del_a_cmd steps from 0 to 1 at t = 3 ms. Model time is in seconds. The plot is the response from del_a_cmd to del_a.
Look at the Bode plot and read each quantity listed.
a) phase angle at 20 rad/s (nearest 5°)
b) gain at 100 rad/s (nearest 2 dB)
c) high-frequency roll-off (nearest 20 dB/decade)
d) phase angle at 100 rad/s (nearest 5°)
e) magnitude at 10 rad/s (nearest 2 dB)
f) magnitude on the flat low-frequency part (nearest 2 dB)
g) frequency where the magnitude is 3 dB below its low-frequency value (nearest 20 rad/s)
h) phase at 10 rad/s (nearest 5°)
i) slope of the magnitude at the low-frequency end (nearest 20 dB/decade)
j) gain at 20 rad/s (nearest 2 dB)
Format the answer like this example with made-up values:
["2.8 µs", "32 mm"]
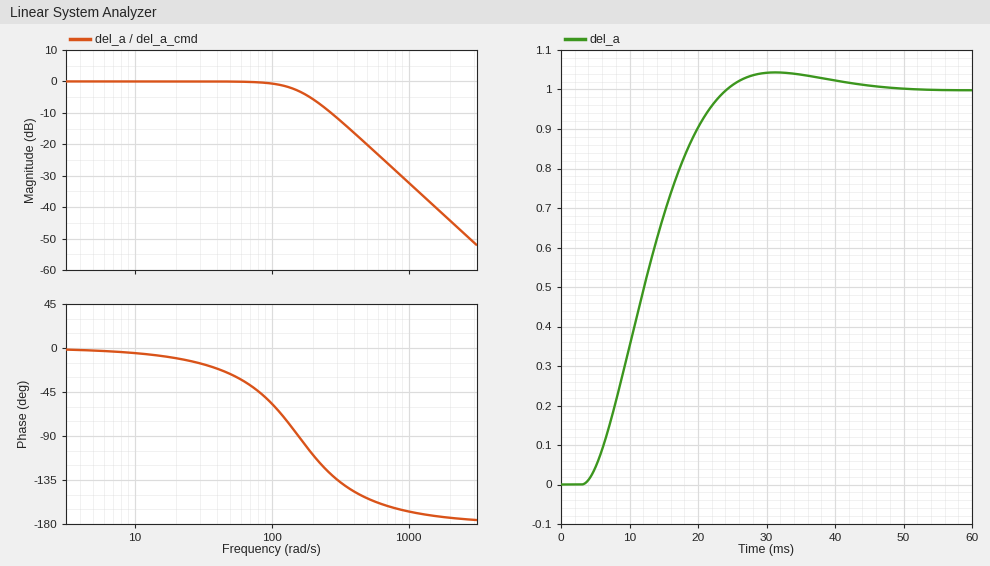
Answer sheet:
["-10°", "0 dB", "-40 dB/decade", "-55°", "0 dB", "0 dB", "160 rad/s", "-5°", "0 dB/decade", "0 dB"]
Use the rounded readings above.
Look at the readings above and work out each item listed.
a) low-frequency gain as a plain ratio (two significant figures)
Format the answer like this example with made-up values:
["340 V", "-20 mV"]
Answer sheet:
["1.0"]
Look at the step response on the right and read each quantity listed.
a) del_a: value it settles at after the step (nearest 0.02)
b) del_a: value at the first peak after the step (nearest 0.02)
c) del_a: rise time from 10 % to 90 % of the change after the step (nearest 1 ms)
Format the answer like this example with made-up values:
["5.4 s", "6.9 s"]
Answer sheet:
["1.00", "1.04", "14 ms"]
